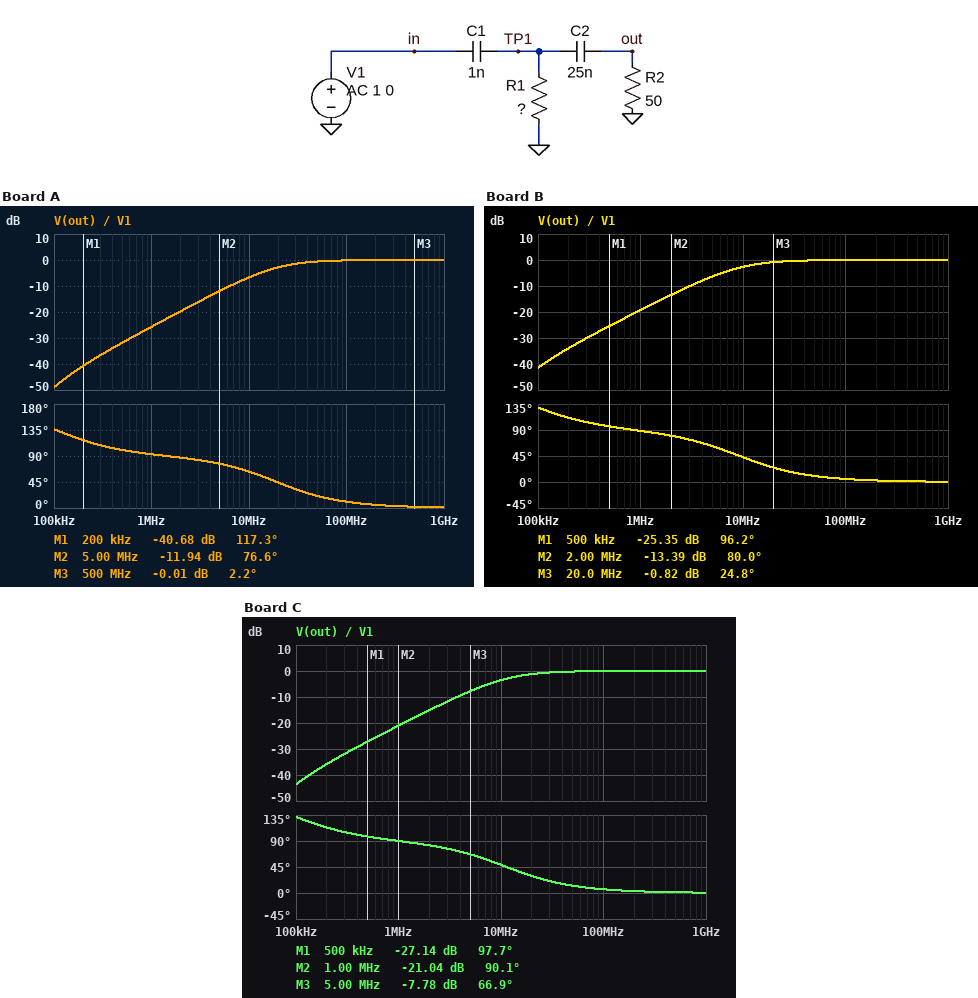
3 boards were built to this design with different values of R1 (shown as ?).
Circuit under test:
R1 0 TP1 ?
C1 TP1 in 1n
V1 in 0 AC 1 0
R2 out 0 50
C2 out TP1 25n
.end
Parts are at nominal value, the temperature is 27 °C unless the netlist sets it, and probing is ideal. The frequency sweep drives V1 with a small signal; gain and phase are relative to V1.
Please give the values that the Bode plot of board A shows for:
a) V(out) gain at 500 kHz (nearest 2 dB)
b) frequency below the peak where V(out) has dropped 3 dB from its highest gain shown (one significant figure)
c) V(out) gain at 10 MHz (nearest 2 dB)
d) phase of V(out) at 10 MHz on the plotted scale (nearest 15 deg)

-32 dB
20 MHz
-6 dB
60 deg
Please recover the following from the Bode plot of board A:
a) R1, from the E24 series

10 Ω
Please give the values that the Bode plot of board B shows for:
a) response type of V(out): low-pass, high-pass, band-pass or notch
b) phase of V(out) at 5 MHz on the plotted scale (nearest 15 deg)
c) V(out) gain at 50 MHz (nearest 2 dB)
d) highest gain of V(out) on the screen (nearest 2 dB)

high-pass
60 deg
0 dB
0 dB
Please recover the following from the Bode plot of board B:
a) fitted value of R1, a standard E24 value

27 Ω
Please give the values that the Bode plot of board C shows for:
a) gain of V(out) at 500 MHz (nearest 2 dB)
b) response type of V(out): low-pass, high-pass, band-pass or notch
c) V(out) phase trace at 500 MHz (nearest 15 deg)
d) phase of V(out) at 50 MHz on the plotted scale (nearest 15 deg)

0 dB
high-pass
0 deg
15 deg
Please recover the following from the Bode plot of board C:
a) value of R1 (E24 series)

20 Ω
